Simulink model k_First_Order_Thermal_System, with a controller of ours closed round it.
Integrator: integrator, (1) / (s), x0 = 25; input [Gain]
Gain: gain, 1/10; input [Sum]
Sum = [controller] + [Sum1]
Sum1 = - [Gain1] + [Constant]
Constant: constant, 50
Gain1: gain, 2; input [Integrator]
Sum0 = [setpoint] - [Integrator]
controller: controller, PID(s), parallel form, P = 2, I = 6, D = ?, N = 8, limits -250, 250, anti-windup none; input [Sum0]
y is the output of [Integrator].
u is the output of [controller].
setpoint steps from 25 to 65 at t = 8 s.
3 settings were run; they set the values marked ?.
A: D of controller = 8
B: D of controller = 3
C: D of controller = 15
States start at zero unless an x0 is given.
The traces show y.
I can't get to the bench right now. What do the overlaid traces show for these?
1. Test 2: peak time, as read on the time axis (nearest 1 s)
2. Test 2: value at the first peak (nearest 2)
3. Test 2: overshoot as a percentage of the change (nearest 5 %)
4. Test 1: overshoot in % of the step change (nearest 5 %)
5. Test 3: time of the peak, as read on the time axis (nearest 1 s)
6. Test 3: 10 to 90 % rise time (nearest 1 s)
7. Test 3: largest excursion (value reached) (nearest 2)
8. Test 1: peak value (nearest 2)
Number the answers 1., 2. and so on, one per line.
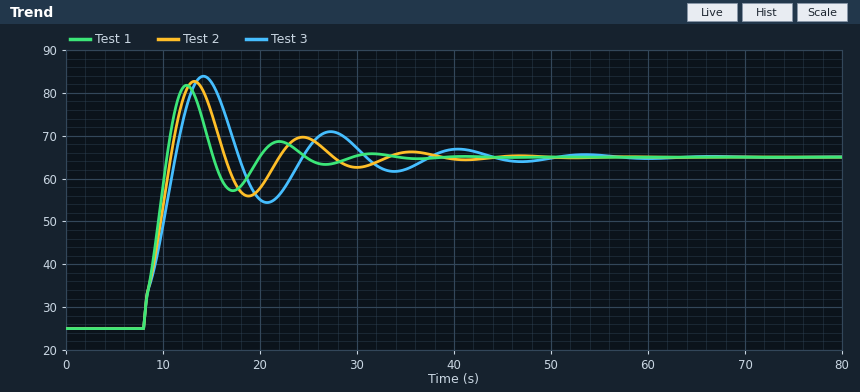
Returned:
1. 13 s
2. 82
3. 45 %
4. 40 %
5. 14 s
6. 3 s
7. 84
8. 82
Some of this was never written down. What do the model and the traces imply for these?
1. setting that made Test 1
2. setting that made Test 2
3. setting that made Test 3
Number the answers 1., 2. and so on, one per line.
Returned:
1. B
2. A
3. C
